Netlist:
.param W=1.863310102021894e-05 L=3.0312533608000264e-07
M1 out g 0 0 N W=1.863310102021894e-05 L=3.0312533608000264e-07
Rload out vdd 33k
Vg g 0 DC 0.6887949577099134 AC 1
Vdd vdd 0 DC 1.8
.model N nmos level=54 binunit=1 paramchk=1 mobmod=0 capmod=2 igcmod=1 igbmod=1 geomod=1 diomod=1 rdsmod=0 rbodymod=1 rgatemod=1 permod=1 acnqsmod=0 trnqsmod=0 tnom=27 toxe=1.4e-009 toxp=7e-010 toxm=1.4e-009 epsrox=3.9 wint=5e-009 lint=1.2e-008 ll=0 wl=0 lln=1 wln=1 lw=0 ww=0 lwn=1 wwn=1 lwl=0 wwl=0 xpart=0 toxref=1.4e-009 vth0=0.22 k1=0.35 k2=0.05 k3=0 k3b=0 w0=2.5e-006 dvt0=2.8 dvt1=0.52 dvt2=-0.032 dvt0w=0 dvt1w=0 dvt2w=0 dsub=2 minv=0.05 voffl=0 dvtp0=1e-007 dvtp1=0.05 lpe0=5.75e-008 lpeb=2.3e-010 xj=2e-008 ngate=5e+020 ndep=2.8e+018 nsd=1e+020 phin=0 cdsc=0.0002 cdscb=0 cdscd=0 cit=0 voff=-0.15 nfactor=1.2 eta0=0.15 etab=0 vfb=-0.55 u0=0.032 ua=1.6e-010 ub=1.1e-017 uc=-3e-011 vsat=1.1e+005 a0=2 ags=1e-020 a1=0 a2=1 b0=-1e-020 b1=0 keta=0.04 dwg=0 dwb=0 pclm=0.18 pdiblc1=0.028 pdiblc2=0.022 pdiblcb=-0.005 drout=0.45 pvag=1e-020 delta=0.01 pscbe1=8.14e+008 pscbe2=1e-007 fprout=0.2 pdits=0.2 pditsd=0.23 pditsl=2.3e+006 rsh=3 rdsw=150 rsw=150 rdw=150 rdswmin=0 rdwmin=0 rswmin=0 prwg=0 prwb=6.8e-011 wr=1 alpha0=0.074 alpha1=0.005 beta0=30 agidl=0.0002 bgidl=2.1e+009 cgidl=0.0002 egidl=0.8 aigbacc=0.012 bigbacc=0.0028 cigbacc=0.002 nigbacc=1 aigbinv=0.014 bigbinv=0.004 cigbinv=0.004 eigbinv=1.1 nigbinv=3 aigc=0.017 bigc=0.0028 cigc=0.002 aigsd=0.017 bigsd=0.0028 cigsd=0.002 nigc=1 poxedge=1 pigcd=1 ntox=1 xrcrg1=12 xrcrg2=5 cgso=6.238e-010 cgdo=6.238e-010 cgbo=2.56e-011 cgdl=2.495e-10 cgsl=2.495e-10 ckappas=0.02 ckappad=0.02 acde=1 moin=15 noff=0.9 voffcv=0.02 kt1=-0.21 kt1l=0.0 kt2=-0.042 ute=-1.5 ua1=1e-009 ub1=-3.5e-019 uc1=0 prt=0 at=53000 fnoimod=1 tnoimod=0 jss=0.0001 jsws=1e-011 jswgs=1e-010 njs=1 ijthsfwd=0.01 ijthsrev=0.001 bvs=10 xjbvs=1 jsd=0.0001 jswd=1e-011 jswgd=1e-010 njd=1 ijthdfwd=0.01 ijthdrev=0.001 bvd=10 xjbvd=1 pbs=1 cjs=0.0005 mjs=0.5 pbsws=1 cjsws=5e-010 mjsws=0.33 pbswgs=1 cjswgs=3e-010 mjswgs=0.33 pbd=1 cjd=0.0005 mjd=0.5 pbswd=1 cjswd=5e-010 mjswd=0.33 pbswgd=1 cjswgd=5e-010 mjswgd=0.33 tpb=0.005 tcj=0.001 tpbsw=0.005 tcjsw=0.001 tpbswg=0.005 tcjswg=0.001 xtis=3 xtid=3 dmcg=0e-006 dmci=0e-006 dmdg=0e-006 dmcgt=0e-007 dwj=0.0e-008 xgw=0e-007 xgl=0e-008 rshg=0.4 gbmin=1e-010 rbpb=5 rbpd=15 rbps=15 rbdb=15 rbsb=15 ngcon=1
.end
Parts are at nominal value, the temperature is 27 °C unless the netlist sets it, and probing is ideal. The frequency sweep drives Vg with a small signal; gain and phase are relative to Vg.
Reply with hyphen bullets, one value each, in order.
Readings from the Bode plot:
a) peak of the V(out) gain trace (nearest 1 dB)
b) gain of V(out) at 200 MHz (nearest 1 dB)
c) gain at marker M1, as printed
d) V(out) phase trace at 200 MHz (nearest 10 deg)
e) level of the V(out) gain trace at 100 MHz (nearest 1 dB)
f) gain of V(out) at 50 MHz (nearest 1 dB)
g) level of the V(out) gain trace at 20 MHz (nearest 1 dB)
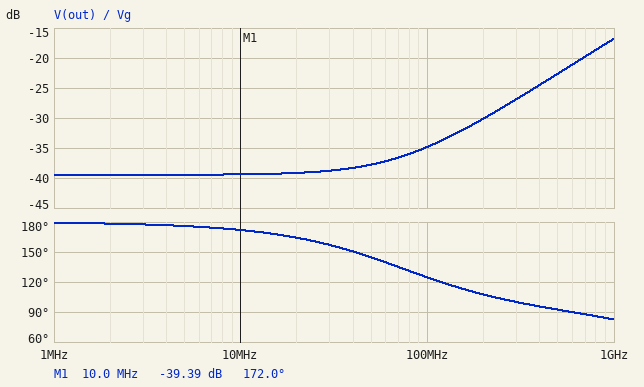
- -17 dB
- -30 dB
- -39.39 dB
- 110 deg
- -35 dB
- -38 dB
- -39 dB
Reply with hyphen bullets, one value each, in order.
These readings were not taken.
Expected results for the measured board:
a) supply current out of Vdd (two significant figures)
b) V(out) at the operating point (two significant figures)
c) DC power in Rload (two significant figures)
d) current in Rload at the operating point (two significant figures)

- 54 µA
- 11 mV
- 97 µW
- 54 µA
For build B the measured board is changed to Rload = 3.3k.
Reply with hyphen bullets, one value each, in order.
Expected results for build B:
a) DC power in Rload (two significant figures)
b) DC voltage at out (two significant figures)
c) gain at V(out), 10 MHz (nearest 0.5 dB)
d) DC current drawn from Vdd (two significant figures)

- 850 µW
- 120 mV
- -13.5 dB
- 510 µA
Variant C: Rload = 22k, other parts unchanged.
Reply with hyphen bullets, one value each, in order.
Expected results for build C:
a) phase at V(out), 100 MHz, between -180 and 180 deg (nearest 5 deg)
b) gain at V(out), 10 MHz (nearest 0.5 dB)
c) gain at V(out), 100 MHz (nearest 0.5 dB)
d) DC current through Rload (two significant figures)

- 135 deg
- -35.5 dB
- -33.0 dB
- 81 µA
